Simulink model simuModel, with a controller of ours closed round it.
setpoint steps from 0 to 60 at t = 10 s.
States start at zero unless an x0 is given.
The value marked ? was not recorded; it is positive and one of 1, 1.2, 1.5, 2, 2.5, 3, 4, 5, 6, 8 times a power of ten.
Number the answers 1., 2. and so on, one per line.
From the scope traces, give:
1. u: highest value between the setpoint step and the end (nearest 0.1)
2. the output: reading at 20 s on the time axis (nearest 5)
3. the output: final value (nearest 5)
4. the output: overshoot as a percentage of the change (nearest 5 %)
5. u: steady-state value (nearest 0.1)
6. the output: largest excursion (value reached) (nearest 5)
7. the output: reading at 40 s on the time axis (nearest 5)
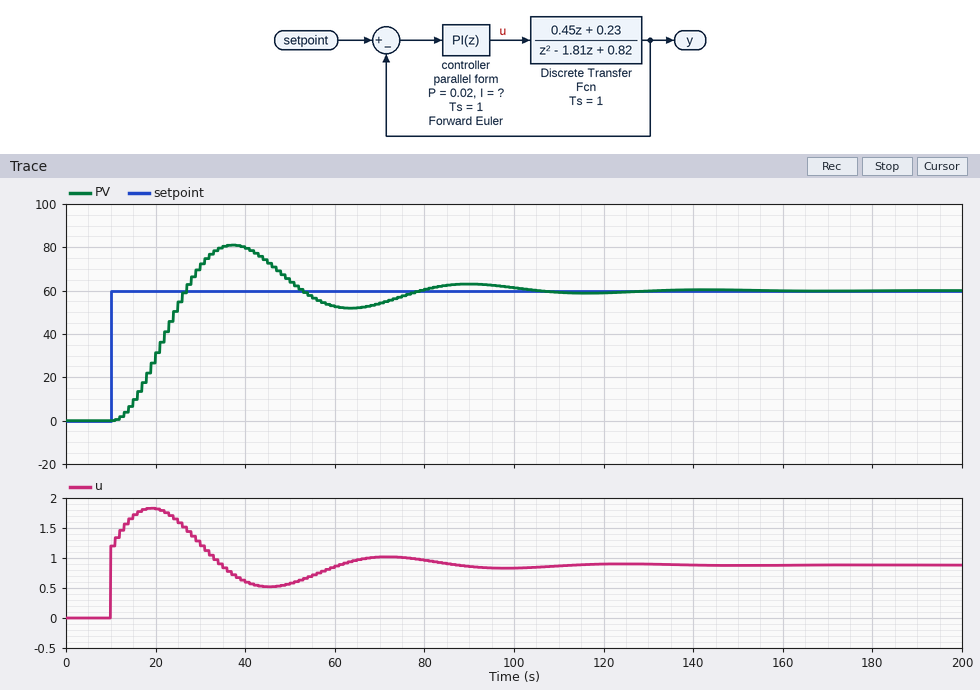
1. 1.8
2. 30
3. 60
4. 35 %
5. 0.9
6. 80
7. 80
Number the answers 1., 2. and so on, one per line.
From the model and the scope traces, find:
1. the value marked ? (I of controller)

1. 0.0025
